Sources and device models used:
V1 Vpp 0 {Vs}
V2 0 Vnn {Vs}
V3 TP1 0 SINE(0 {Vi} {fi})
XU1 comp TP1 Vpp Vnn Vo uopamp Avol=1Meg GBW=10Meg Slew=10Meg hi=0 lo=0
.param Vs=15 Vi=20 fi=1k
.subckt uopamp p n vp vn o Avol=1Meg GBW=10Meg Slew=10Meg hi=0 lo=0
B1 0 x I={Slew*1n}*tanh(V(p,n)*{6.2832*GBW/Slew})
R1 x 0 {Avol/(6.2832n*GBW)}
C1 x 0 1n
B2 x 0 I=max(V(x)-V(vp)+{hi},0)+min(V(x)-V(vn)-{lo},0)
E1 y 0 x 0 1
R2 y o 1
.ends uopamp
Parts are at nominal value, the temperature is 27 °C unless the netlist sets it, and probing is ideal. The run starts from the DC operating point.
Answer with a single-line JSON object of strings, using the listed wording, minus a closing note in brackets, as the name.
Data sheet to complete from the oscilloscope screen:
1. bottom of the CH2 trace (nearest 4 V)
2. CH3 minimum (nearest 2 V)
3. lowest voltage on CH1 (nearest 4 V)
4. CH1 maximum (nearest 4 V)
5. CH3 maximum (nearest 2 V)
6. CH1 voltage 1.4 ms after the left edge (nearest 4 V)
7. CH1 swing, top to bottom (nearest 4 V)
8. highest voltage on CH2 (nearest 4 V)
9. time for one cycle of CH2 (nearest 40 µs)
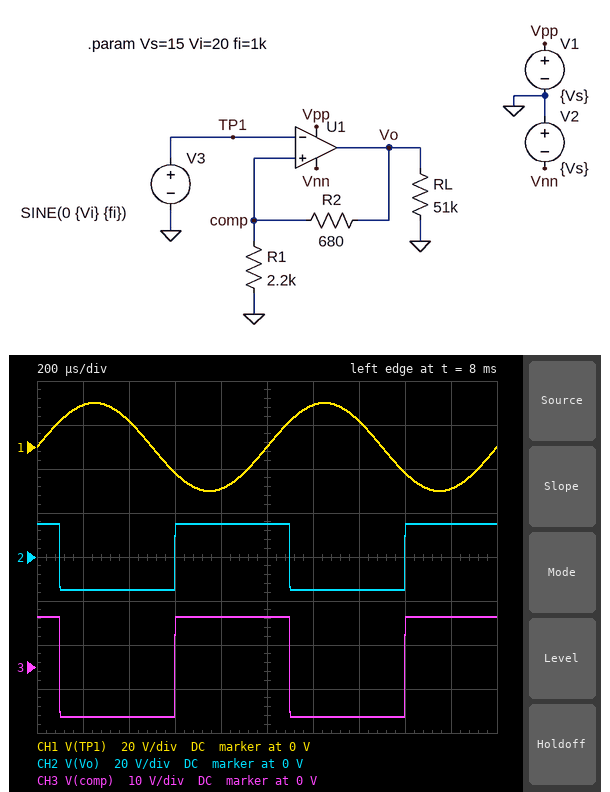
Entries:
{"bottom of the CH2 trace": "-16 V", "CH3 minimum": "-12 V", "lowest voltage on CH1": "-20 V", "CH1 maximum": "20 V", "CH3 maximum": "12 V", "CH1 voltage 1.4 ms after the left edge": "12 V", "CH1 swing, top to bottom": "40 V", "highest voltage on CH2": "16 V", "time for one cycle of CH2": "1.00 ms"}
